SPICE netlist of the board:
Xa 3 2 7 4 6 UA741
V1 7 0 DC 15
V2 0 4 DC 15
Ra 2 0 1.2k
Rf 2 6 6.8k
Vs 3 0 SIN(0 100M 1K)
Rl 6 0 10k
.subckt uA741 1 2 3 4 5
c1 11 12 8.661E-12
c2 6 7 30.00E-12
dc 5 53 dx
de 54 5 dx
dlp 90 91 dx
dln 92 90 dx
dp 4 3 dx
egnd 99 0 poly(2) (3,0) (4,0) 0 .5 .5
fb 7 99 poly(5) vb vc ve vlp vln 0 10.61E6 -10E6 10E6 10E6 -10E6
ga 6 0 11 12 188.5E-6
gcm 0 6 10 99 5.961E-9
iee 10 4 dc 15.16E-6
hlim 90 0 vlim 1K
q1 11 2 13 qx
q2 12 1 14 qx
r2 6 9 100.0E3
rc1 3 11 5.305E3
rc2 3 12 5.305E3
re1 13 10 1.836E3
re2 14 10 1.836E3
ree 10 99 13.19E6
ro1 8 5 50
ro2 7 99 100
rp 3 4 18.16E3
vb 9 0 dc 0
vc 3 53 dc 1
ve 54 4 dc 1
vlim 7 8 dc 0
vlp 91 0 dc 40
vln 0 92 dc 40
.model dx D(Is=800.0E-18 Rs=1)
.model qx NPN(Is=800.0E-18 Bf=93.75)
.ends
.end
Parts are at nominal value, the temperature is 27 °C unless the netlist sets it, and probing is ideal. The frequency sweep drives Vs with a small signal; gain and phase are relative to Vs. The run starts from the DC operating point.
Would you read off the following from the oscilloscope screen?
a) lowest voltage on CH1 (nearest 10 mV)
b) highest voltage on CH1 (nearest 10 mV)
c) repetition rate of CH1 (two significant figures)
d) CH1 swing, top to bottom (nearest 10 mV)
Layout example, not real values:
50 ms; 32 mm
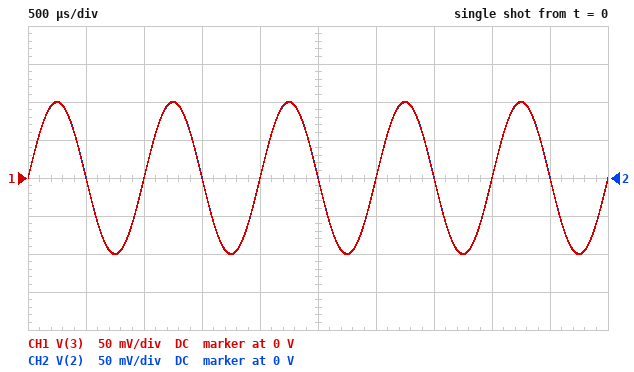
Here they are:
-100 mV; 100 mV; 1.0 kHz; 200 mV
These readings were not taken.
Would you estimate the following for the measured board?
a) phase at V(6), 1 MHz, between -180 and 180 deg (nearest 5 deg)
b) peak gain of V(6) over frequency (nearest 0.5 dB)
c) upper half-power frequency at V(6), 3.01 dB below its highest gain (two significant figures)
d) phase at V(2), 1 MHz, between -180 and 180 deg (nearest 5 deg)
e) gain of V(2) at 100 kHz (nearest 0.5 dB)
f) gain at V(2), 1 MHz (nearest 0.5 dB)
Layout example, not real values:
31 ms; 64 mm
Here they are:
-115 deg; 16.5 dB; 160 kHz; -115 deg; -1.5 dB; -17.5 dB
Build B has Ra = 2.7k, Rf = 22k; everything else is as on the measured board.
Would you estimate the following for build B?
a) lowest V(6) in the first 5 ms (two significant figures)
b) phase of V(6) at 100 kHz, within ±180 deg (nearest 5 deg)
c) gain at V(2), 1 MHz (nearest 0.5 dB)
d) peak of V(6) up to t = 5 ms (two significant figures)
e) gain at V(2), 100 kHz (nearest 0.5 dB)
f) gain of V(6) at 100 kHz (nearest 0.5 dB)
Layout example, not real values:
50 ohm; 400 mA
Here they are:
-910 mV; -45 deg; -20.5 dB; 920 mV; -2.5 dB; 17.0 dB
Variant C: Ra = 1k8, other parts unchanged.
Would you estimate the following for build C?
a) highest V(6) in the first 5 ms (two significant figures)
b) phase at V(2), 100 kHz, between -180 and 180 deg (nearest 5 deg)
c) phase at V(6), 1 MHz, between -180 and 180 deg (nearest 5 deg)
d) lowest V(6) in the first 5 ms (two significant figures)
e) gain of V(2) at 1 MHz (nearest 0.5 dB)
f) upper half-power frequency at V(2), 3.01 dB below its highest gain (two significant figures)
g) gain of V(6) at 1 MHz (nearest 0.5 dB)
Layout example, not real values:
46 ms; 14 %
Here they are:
480 mV; -25 deg; -110 deg; -480 mV; -14.5 dB; 230 kHz; -0.5 dB
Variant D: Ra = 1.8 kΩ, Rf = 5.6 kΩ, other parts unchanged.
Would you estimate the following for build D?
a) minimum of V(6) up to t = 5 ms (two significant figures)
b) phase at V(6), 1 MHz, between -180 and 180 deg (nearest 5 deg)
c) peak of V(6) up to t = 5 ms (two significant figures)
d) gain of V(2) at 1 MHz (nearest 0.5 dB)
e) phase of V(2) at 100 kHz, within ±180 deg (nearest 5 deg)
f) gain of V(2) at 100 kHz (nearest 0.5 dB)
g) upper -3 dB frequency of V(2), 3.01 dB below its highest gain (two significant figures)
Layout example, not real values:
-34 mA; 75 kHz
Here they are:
-410 mV; -110 deg; 410 mV; -13.0 dB; -25 deg; -0.5 dB; 280 kHz
